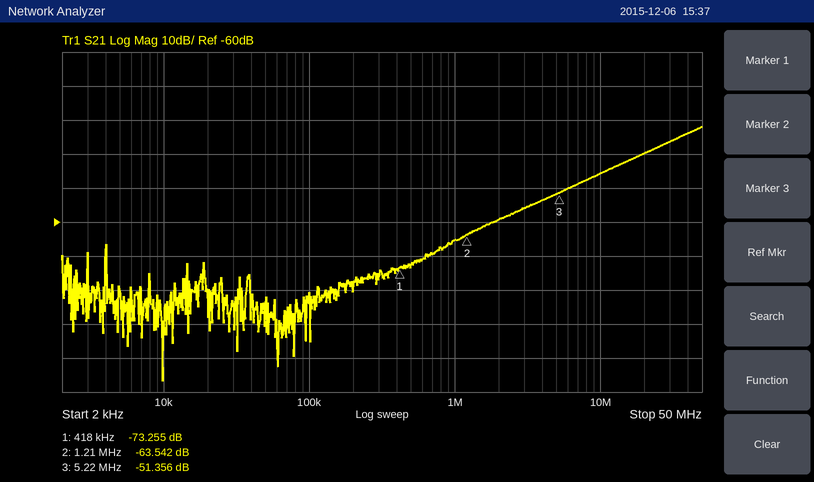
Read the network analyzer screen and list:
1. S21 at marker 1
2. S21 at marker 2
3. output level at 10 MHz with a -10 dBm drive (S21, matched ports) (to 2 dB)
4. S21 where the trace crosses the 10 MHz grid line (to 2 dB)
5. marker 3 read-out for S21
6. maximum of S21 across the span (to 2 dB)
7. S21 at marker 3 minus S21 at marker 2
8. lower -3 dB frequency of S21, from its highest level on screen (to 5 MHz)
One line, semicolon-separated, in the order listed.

-73.255 dB; -63.542 dB; -56 dBm; -46 dB; -51.356 dB; -32 dB; 12.186 dB; 35 MHz
